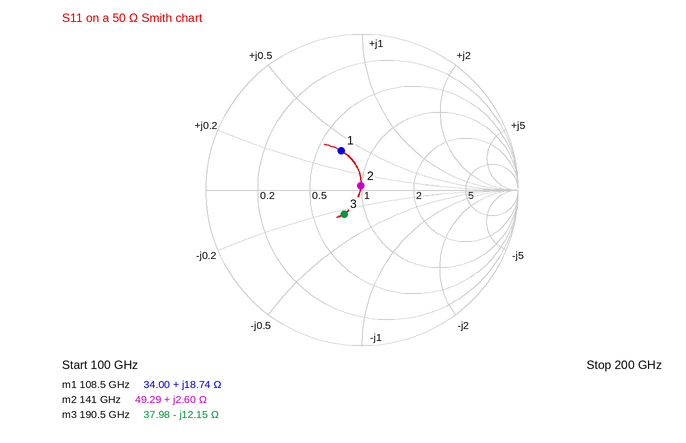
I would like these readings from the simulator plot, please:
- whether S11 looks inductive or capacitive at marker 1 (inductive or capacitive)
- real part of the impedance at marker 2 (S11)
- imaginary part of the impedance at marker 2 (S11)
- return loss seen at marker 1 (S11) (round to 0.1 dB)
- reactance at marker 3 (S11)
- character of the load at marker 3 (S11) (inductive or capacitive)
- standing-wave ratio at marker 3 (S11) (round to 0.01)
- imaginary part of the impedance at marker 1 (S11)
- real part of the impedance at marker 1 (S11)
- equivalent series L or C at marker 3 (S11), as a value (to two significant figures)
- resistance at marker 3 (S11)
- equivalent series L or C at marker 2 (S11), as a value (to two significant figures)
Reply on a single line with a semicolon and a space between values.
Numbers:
inductive; 49.29 Ω; +2.60 Ω; 10.9 dB; -12.15 Ω; capacitive; 1.48; +18.74 Ω; 34.00 Ω; 69 fF; 37.98 Ω; 2.9 pH
